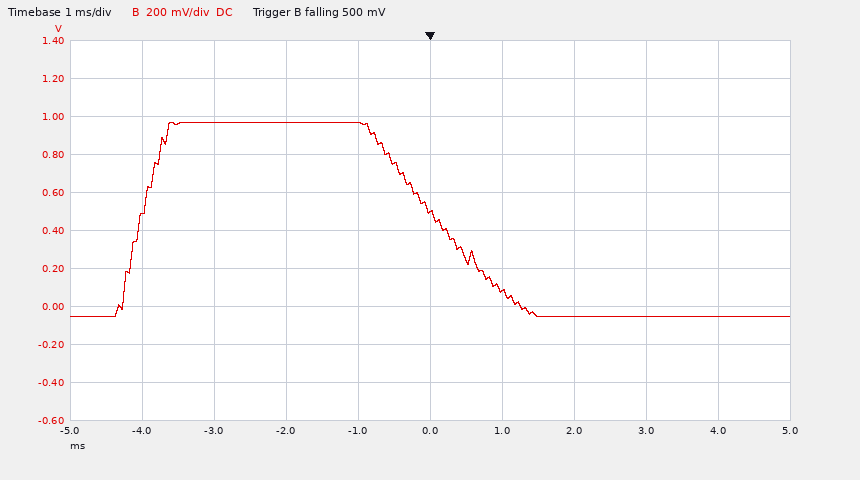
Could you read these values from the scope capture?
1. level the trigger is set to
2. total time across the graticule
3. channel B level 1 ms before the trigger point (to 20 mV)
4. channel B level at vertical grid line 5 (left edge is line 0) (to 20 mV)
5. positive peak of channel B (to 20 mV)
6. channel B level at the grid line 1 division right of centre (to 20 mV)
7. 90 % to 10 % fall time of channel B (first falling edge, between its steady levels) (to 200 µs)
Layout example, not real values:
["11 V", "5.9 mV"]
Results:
["500 mV", "10 ms", "960 mV", "500 mV", "960 mV", "80 mV", "1.8 ms"]
